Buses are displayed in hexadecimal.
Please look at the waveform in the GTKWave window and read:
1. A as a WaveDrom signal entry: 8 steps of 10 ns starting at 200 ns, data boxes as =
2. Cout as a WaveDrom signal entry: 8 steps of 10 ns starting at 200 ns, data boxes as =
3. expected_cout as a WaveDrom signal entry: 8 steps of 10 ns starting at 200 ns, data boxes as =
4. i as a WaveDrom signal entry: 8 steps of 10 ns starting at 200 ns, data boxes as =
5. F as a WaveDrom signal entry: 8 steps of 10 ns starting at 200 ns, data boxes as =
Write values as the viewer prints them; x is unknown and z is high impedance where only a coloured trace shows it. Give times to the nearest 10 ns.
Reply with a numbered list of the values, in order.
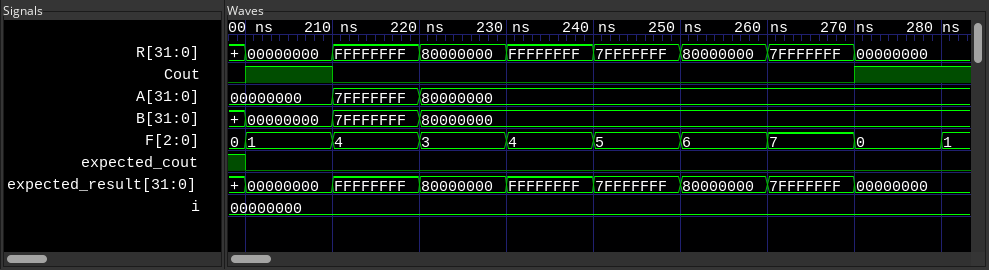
1. {name: 'A', wave: '===.....', data: '00000000 7FFFFFFF 80000000'}
2. {name: 'Cout', wave: '10.....1'}
3. {name: 'expected_cout', wave: '0.......'}
4. {name: 'i', wave: '=.......', data: '00000000'}
5. {name: 'F', wave: '========', data: '1 4 3 4 5 6 7 0'}
